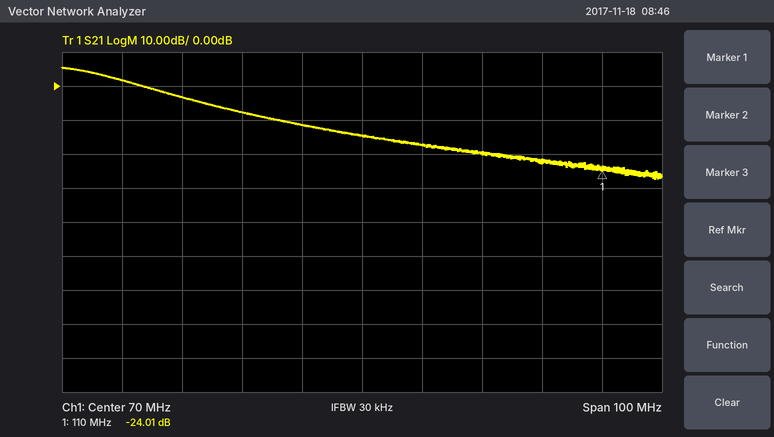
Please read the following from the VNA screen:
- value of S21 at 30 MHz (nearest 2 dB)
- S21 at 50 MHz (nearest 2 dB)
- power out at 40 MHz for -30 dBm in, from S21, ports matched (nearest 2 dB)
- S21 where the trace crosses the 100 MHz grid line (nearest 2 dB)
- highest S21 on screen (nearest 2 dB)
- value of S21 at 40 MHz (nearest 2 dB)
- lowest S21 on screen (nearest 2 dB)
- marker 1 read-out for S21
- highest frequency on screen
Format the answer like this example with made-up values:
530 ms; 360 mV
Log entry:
2 dB; -8 dB; -34 dBm; -22 dB; 6 dB; -4 dB; -28 dB; -24.01 dB; 120 MHz
